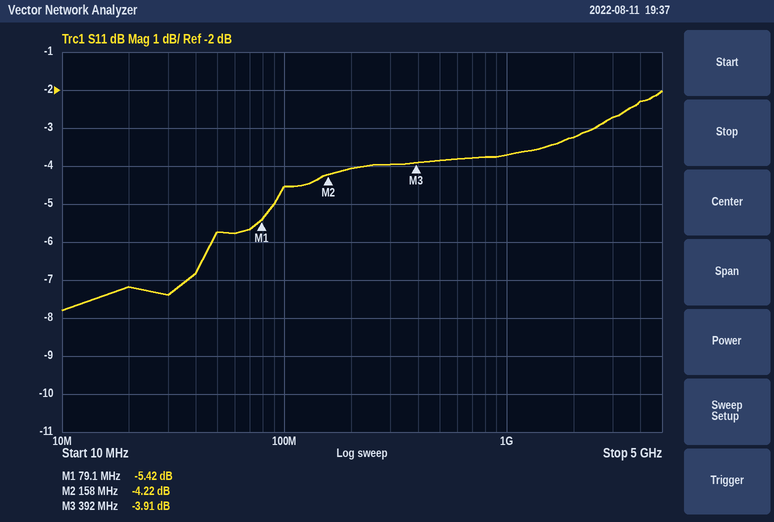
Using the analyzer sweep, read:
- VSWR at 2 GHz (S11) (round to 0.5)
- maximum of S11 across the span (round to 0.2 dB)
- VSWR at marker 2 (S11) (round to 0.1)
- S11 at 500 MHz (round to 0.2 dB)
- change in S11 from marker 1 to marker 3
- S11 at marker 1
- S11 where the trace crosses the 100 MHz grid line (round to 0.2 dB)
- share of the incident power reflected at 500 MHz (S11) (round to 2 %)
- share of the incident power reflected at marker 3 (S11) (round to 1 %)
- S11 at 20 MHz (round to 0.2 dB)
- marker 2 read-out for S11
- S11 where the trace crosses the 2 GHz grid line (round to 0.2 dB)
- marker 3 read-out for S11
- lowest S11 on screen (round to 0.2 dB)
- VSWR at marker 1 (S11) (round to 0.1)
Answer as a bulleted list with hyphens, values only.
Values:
- 5.5
- -2.0 dB
- 4.2
- -3.8 dB
- 1.51 dB
- -5.42 dB
- -4.6 dB
- 42 %
- 41 %
- -7.2 dB
- -4.22 dB
- -3.2 dB
- -3.91 dB
- -7.8 dB
- 3.3
